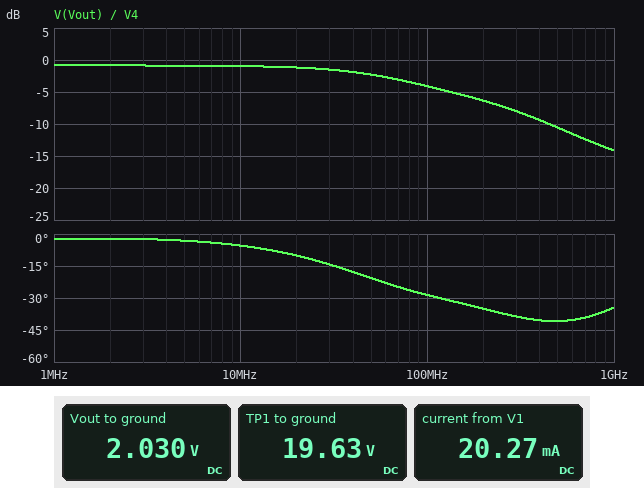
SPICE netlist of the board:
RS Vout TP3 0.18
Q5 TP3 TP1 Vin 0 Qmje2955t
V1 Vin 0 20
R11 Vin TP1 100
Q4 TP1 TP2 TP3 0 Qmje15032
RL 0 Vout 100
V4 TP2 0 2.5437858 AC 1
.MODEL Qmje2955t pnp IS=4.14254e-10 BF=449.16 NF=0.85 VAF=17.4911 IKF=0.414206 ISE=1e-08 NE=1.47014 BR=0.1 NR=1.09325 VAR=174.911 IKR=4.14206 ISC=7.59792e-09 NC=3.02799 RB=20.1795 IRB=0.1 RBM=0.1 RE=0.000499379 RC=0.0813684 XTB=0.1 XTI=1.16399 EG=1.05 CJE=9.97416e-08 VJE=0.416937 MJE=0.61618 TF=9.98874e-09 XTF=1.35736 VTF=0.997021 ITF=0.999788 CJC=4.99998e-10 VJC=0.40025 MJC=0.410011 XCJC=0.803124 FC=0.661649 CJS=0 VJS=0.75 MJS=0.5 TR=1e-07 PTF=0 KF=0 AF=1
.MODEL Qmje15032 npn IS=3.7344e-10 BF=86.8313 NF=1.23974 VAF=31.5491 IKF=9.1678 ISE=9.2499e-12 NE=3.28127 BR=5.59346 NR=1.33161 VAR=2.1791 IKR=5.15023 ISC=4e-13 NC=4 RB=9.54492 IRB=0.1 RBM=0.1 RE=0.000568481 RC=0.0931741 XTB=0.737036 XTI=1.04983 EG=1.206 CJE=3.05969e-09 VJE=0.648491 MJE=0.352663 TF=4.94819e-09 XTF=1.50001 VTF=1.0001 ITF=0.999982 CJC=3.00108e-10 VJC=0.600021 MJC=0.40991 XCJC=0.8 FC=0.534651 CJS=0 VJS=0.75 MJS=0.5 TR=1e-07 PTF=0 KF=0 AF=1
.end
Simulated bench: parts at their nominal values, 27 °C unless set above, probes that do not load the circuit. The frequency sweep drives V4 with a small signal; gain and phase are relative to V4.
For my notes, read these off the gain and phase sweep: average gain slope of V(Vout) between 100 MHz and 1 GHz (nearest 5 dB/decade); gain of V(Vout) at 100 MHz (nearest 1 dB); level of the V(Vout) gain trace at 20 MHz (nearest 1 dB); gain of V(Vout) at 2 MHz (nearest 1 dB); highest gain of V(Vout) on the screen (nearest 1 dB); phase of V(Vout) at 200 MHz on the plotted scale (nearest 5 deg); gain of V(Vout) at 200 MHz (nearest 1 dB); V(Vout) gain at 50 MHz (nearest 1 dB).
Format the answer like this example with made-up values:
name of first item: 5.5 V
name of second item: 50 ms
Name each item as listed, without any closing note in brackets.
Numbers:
average gain slope of V(Vout) between 100 MHz and 1 GHz: -10 dB/decade
gain of V(Vout) at 100 MHz: -4 dB
level of the V(Vout) gain trace at 20 MHz: -1 dB
gain of V(Vout) at 2 MHz: -1 dB
highest gain of V(Vout) on the screen: -1 dB
phase of V(Vout) at 200 MHz on the plotted scale: -35 deg
gain of V(Vout) at 200 MHz: -6 dB
V(Vout) gain at 50 MHz: -2 dB
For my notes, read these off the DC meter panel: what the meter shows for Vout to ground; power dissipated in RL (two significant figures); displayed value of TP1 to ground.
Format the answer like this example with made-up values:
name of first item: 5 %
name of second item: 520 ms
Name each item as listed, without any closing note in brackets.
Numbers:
what the meter shows for Vout to ground: 2.030 V
power dissipated in RL: 41 mW
displayed value of TP1 to ground: 19.63 V
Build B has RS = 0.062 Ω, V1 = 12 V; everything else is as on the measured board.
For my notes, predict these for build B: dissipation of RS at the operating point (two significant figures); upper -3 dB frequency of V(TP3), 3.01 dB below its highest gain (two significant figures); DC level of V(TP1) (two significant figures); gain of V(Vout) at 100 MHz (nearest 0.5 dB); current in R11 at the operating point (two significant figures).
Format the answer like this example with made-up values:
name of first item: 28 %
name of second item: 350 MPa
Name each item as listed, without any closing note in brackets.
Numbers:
dissipation of RS at the operating point: 25 µW
upper -3 dB frequency of V(TP3), 3.01 dB below its highest gain: 54 MHz
DC level of V(TP1): 12 V
gain of V(Vout) at 100 MHz: -5.0 dB
current in R11 at the operating point: 3.8 mA
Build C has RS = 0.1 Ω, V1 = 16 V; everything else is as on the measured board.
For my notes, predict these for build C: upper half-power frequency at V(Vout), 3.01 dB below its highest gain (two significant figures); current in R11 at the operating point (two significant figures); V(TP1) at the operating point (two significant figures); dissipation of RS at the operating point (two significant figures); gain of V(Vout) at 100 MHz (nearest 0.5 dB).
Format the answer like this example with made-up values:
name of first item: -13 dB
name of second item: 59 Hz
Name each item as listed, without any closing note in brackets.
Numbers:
upper half-power frequency at V(Vout), 3.01 dB below its highest gain: 62 MHz
current in R11 at the operating point: 3.8 mA
V(TP1) at the operating point: 16 V
dissipation of RS at the operating point: 41 µW
gain of V(Vout) at 100 MHz: -4.5 dB
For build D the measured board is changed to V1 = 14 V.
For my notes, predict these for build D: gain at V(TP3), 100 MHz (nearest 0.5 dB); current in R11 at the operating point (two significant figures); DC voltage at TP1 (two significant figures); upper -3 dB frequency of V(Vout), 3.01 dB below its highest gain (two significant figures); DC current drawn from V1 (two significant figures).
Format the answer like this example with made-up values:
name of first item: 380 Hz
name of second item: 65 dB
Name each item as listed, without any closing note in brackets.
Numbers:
gain at V(TP3), 100 MHz: -4.5 dB
current in R11 at the operating point: 3.8 mA
DC voltage at TP1: 14 V
upper -3 dB frequency of V(Vout), 3.01 dB below its highest gain: 58 MHz
DC current drawn from V1: 20 mA
